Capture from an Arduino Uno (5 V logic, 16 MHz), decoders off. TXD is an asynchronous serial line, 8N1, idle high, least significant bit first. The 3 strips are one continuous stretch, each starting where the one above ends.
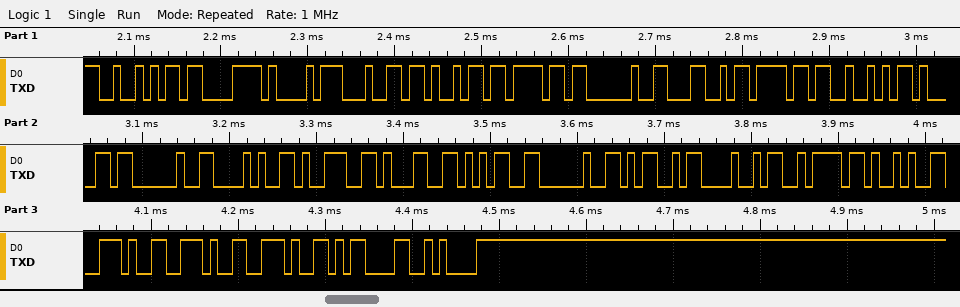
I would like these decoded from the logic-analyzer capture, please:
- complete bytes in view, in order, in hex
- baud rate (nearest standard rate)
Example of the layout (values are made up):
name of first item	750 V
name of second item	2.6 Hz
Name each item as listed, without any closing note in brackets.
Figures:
complete bytes in view, in order, in hex	52 C3 A1 64 69 6F 20 4C 6F 52 61 20 28 39 31 35 20 4D 48 7A 29 2E 2E 2E 0D 0A
baud rate	115200 baud
